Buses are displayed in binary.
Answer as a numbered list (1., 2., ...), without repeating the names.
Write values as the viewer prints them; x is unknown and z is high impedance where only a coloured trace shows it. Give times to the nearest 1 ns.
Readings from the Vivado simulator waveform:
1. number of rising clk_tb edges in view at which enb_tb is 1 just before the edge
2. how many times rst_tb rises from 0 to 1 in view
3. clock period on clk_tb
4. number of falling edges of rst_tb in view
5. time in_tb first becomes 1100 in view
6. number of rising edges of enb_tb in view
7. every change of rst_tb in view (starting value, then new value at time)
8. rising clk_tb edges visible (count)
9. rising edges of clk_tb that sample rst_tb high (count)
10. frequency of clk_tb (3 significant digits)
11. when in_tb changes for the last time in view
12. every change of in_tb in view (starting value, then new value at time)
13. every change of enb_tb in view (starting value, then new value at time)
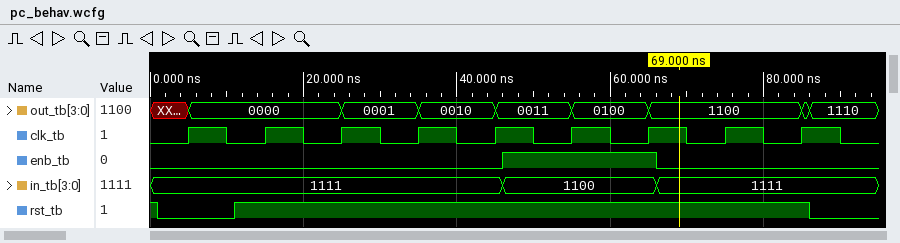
1. 2
2. 1
3. 10 ns
4. 2
5. 46 ns
6. 1
7. 1, 0 at 1 ns, 1 at 11 ns, 0 at 86 ns
8. 9
9. 8
10. 100 MHz
11. 66 ns
12. 1111, 1100 at 46 ns, 1111 at 66 ns
13. 0, 1 at 46 ns, 0 at 66 ns
